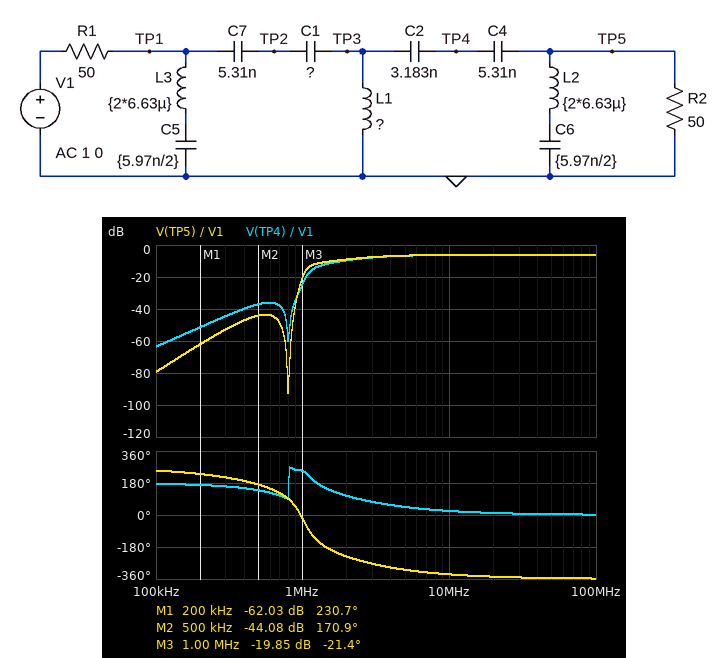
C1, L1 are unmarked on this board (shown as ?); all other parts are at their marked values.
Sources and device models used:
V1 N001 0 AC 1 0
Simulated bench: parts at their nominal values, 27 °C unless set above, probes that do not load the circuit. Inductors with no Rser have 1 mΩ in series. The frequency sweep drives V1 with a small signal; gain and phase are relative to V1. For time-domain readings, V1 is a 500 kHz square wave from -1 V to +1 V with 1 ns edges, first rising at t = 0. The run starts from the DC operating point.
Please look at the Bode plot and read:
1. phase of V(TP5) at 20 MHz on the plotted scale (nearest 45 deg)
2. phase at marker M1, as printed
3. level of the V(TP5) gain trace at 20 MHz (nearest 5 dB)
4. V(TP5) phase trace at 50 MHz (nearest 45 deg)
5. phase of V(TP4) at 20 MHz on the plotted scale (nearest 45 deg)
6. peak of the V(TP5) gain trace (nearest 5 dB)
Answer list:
-360 deg
230.7 deg
-5 dB
-360 deg
0 deg
-5 dB
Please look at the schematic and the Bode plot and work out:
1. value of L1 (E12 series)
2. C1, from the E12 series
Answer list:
1.5 µH
6.8 nF
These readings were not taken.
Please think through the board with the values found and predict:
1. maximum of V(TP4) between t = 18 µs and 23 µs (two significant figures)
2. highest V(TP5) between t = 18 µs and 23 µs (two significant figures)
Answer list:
1.0 V
1.0 V
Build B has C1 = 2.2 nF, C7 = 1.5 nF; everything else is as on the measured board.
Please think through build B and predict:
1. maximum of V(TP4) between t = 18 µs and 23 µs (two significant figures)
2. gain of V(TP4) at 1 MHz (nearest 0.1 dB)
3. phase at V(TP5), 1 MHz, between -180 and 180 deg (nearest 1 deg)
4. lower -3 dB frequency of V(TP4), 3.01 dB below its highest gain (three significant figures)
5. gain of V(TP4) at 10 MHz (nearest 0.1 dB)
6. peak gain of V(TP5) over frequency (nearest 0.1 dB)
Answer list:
980 mV
-39.8 dB
7 deg
2.66 MHz
-6.1 dB
-6.0 dB
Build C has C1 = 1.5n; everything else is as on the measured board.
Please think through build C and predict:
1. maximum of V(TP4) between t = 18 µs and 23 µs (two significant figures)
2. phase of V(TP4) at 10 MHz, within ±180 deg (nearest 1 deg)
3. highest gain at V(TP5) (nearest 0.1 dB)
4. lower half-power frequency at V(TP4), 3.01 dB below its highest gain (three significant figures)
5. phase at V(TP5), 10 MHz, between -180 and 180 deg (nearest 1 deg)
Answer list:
980 mV
28 deg
-6.0 dB
2.39 MHz
31 deg
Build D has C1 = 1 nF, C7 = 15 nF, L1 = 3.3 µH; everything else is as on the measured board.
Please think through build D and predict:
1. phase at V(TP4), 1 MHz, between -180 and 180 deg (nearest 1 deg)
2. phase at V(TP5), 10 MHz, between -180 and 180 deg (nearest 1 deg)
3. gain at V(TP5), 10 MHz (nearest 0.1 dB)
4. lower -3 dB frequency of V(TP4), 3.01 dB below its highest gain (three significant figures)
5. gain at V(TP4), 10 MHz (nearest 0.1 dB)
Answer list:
-90 deg
25 deg
-6.0 dB
1.65 MHz
-6.1 dB
